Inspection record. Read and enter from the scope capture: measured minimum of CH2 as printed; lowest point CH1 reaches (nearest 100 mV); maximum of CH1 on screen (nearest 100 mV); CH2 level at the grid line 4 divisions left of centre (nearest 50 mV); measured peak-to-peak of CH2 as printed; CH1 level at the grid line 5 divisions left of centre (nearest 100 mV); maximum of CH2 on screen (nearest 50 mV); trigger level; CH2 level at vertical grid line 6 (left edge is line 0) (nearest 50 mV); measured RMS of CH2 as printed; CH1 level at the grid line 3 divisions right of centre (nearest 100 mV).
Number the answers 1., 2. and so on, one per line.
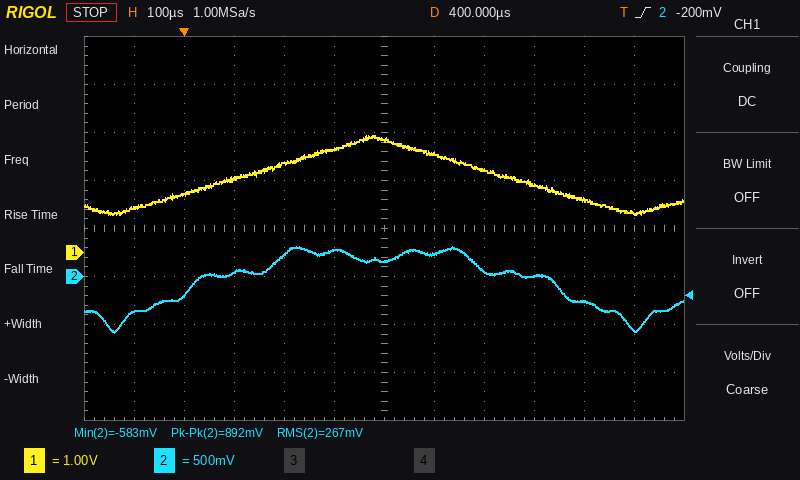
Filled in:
1. -583 mV
2. 800 mV
3. 2.4 V
4. -200 mV
5. 892 mV
6. 900 mV
7. 300 mV
8. -200 mV
9. 150 mV
10. 267 mV
11. 1.4 V
